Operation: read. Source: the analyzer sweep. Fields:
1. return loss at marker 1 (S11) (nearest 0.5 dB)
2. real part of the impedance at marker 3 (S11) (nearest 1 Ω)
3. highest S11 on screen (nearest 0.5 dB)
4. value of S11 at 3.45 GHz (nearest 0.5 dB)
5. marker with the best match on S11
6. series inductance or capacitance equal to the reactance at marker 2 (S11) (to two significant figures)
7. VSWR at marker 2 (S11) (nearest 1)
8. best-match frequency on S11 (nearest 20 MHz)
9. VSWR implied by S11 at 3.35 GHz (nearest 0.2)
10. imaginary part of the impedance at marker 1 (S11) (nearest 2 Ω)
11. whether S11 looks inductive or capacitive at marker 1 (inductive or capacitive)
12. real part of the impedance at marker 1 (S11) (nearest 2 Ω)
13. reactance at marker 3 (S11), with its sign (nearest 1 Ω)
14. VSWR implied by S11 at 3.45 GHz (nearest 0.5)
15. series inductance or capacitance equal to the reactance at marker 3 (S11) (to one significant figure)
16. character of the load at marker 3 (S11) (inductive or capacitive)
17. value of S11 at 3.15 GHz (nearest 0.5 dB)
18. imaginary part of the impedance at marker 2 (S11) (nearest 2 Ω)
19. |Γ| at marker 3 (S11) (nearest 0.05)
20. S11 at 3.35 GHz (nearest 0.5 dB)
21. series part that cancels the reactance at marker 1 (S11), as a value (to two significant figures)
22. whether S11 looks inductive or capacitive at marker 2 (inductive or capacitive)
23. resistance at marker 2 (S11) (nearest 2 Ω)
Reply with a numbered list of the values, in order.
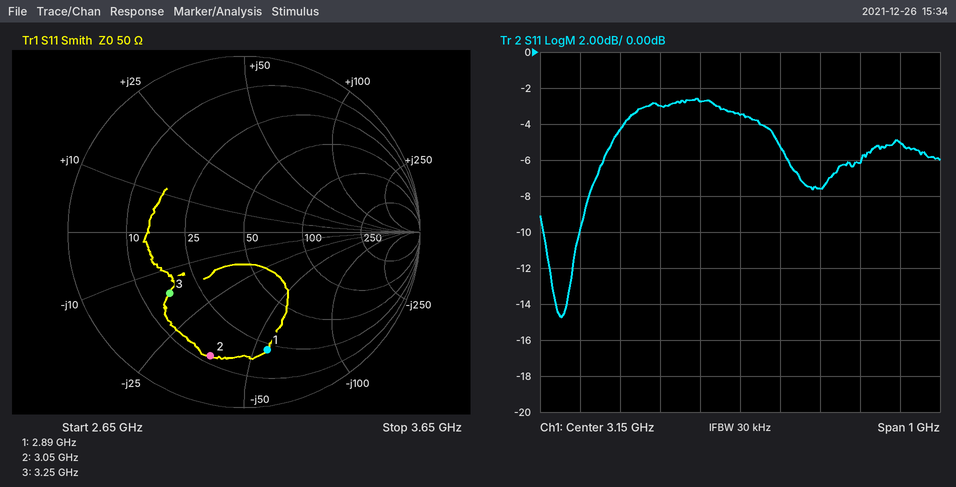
1. 3.5 dB
2. 16 Ω
3. -2.5 dB
4. -6.0 dB
5. marker 3
6. 1.4 pF
7. 6
8. 2.70 GHz
9. 2.4
10. -56 Ω
11. capacitive
12. 22 Ω
13. -16 Ω
14. 3.0
15. 3 pF
16. capacitive
17. -3.5 dB
18. -36 Ω
19. 0.55
20. -7.5 dB
21. 3.1 nH
22. capacitive
23. 12 Ω
